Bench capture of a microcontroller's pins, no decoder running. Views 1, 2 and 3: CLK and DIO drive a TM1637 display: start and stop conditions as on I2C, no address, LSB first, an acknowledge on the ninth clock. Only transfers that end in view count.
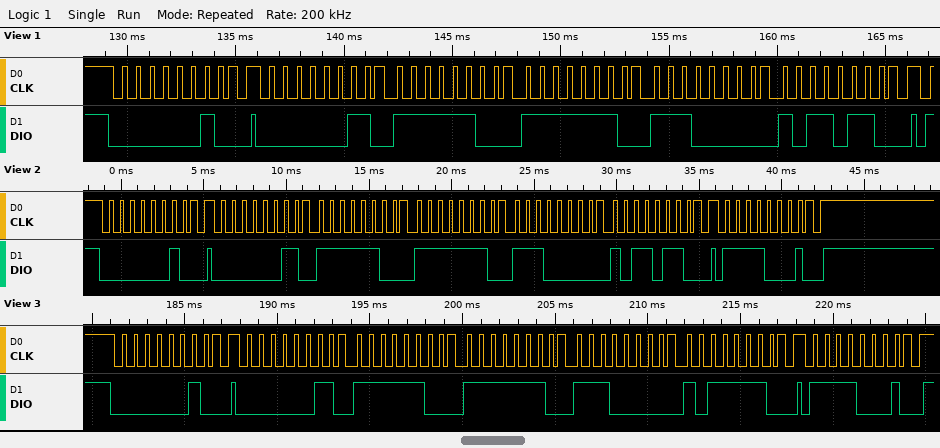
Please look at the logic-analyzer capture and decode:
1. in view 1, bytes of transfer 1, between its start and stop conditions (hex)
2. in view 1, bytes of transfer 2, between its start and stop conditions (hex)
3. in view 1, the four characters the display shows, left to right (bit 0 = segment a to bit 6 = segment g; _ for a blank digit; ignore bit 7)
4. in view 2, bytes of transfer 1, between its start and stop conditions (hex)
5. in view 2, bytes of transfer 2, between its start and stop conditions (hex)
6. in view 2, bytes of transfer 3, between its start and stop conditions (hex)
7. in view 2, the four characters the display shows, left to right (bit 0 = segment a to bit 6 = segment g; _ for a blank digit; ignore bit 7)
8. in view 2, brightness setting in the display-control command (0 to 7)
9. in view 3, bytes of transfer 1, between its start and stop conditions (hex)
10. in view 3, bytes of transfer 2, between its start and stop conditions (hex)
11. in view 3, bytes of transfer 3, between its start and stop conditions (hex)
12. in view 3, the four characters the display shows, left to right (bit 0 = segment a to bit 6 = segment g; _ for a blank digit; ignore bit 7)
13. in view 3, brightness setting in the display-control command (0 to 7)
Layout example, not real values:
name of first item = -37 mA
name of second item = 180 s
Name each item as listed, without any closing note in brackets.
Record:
in view 1, bytes of transfer 1, between its start and stop conditions = 40
in view 1, bytes of transfer 2, between its start and stop conditions = C0 3F 7F 07 6D
in view 1, the four characters the display shows, left to right = 0875
in view 2, bytes of transfer 1, between its start and stop conditions = 40
in view 2, bytes of transfer 2, between its start and stop conditions = C0 3F 7F 07 6D
in view 2, bytes of transfer 3, between its start and stop conditions = 8F
in view 2, the four characters the display shows, left to right = 0875
in view 2, brightness setting in the display-control command = 7
in view 3, bytes of transfer 1, between its start and stop conditions = 40
in view 3, bytes of transfer 2, between its start and stop conditions = C0 3F 7F 07 7D
in view 3, bytes of transfer 3, between its start and stop conditions = 8F
in view 3, the four characters the display shows, left to right = 0876
in view 3, brightness setting in the display-control command = 7
